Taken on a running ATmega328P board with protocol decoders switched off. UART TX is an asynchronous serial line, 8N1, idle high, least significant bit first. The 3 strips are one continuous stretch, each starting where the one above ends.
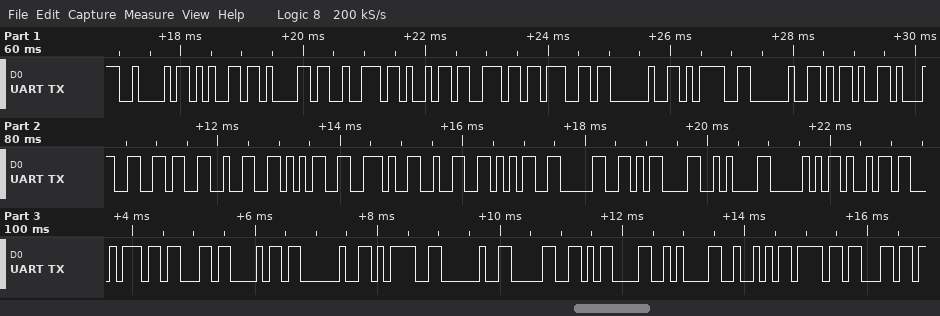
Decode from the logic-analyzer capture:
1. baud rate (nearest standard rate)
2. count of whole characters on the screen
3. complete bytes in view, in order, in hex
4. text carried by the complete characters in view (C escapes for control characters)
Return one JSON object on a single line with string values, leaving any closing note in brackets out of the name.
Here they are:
{"baud rate": "9600 baud", "count of whole characters on the screen": "35", "complete bytes in view, in order, in hex": "42 65 61 72 69 6E 67 20 3D 20 2D 31 36 32 35 2E 32 35 30 0D 0A 50 69 74 63 68 20 3D 20 30 0D 0A 52 6F 6C", "text carried by the complete characters in view": "\"Bearing = -1625.250\\r\\nPitch = 0\\r\\nRol\""}
